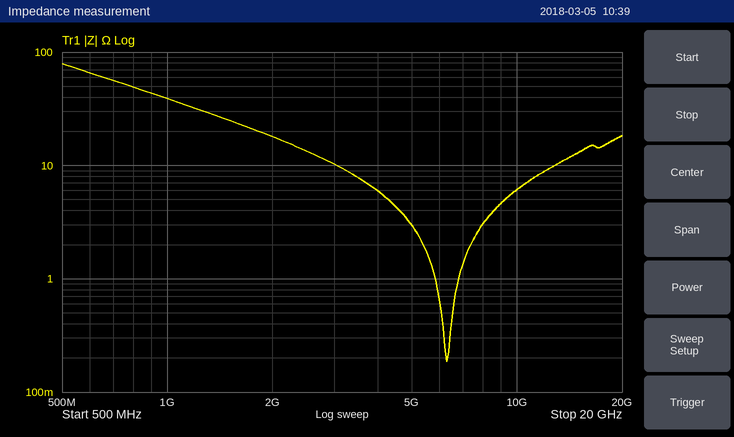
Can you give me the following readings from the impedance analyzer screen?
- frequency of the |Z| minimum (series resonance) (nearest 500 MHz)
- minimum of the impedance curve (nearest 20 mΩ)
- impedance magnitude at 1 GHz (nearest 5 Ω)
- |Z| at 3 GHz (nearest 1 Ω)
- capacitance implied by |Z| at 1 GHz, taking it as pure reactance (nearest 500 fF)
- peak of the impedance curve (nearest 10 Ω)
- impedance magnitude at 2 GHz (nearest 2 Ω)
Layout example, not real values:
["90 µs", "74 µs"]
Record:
["6.5 GHz", "180 mΩ", "40 Ω", "10 Ω", "4.0 pF", "80 Ω", "18 Ω"]
